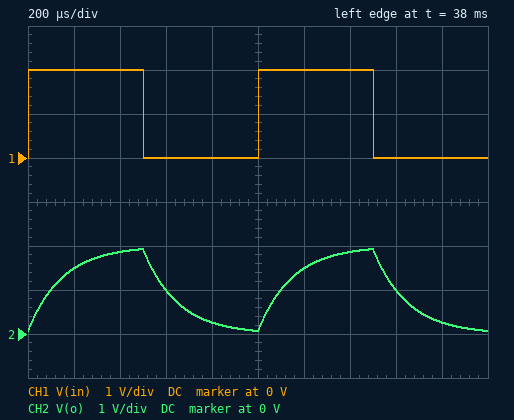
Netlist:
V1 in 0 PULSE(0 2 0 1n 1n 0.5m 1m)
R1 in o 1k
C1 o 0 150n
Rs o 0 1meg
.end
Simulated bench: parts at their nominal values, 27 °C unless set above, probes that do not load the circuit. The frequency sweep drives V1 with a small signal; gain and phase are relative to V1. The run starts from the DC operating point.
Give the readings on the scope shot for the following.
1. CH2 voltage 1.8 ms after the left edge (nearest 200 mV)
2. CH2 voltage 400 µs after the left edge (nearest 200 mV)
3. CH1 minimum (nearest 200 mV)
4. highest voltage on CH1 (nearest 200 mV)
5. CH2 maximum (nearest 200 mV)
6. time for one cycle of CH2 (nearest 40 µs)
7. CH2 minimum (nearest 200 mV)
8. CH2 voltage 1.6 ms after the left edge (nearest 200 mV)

200 mV
1.8 V
0 V
2.0 V
2.0 V
1.00 ms
0 V
1.0 V
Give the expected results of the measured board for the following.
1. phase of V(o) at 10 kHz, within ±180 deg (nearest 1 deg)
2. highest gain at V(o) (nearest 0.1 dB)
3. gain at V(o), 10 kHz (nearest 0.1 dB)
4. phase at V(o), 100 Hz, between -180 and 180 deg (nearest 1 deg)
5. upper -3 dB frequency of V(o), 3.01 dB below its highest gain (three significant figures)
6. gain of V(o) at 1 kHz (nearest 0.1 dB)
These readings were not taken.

-84 deg
0 dB
-19.5 dB
-5 deg
1.06 kHz
-2.8 dB
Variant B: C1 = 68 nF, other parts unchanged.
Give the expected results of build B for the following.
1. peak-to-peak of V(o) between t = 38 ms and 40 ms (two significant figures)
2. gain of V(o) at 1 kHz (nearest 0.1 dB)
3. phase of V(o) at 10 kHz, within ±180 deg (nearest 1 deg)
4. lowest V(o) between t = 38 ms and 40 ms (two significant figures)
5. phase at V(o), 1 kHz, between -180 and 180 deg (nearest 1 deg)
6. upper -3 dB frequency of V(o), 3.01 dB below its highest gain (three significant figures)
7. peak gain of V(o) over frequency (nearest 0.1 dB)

2.0 V
-0.7 dB
-77 deg
1.3 mV
-23 deg
2.34 kHz
0 dB
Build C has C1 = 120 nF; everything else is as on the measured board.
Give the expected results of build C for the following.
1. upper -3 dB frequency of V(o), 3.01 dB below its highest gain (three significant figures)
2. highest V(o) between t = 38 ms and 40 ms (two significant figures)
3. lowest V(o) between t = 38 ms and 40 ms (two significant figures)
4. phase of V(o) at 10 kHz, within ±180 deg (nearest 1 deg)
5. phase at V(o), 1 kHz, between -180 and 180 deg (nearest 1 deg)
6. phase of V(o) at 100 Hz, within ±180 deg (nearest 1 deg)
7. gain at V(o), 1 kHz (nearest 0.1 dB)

1.33 kHz
2.0 V
30 mV
-82 deg
-37 deg
-4 deg
-2.0 dB
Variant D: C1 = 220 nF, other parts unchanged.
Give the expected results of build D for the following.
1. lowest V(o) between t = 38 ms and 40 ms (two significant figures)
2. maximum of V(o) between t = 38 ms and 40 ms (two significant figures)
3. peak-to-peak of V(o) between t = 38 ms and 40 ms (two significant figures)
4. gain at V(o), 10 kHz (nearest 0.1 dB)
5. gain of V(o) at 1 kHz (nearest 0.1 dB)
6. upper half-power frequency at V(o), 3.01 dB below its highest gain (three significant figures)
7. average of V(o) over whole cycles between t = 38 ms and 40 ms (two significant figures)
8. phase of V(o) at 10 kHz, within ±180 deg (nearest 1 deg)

190 mV
1.8 V
1.6 V
-22.8 dB
-4.6 dB
724 Hz
1.0 V
-86 deg
